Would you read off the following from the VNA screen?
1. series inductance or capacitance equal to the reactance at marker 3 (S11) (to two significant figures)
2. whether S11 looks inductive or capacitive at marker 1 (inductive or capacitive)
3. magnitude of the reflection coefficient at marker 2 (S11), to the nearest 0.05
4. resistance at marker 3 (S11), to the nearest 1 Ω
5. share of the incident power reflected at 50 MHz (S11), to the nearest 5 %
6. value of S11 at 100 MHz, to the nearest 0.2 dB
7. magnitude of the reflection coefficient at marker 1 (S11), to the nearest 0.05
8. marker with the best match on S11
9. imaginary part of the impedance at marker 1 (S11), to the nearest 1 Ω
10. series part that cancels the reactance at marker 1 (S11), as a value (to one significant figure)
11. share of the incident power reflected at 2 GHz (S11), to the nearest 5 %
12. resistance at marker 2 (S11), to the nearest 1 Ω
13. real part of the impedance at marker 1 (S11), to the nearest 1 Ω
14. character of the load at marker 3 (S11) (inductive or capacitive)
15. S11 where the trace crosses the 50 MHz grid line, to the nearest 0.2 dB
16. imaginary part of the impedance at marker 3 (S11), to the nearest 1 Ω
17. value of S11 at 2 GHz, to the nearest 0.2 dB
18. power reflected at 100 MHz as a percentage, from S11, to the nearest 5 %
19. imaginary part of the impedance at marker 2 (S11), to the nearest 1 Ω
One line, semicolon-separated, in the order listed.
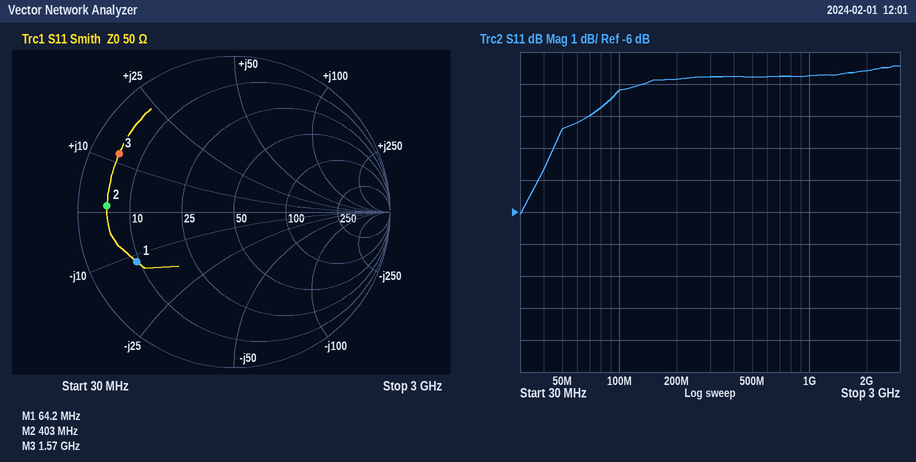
1.2 nH; capacitive; 0.80; 5 Ω; 45 %; -2.2 dB; 0.70; marker 1; -12 Ω; 30 nH; 70 %; 5 Ω; 9 Ω; inductive; -3.4 dB; +12 Ω; -1.6 dB; 60 %; +1 Ω
